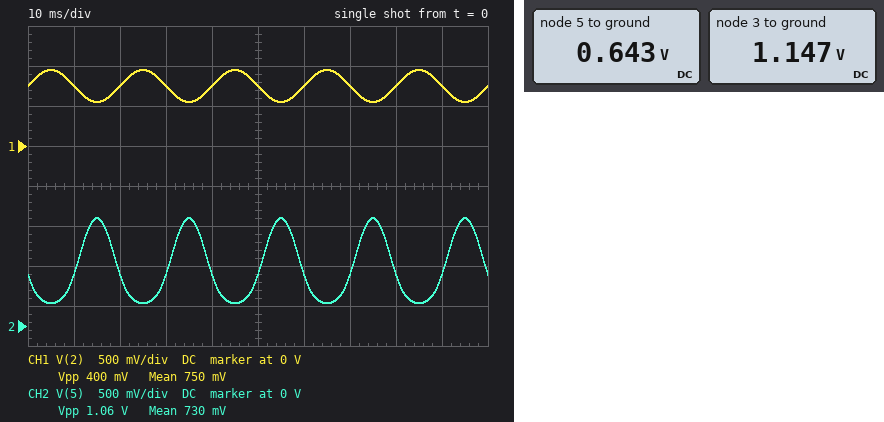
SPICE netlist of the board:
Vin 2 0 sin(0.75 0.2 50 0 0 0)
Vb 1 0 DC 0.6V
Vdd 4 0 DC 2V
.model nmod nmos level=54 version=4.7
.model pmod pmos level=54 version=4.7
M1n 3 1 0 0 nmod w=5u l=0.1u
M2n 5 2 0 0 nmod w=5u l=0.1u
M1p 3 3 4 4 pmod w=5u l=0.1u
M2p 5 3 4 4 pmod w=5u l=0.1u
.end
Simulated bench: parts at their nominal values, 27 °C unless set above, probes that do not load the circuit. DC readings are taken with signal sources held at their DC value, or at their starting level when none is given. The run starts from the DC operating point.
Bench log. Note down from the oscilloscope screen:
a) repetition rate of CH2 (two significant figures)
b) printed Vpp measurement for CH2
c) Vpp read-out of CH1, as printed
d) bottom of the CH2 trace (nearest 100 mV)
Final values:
50 Hz
1.06 V
400 mV
300 mV
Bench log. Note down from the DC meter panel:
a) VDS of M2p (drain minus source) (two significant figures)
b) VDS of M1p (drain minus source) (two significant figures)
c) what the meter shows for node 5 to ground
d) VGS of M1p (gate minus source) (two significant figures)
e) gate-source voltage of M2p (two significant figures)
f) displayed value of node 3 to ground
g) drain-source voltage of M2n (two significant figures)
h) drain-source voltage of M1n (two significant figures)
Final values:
-1.4 V
-850 mV
0.643 V
-850 mV
-850 mV
1.147 V
640 mV
1.1 V
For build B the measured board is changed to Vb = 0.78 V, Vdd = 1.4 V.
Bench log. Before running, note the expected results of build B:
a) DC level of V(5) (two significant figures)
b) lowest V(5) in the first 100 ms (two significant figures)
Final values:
540 mV
250 mV
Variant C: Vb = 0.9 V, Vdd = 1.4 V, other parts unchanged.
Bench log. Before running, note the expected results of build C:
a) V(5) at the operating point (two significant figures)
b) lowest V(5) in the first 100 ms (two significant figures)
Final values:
680 mV
330 mV
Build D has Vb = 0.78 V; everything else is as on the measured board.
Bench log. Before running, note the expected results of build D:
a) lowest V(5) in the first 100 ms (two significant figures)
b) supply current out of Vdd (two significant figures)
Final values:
550 mV
3.4 mA
